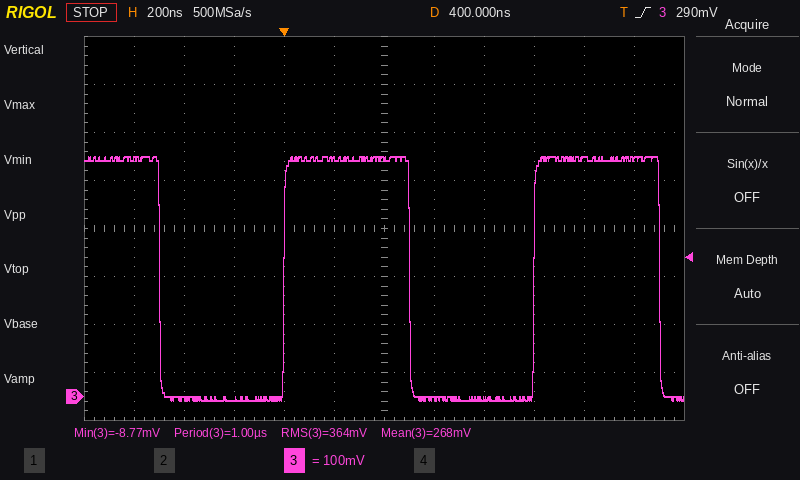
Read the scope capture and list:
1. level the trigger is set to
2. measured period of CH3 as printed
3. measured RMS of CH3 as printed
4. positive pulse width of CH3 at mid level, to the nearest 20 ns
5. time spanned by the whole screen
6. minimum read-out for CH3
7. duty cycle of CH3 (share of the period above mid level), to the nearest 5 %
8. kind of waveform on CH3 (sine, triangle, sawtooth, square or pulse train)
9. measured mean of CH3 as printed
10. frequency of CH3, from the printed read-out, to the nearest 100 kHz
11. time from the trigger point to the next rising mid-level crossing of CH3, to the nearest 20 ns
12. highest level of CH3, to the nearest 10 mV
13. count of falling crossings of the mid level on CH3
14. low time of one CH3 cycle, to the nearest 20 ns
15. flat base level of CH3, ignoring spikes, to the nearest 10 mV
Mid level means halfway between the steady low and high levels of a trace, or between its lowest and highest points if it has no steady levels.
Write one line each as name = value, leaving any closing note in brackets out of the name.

level the trigger is set to = 290 mV
measured period of CH3 as printed = 1.00 µs
measured RMS of CH3 as printed = 364 mV
positive pulse width of CH3 at mid level, to the nearest 20 ns = 500 ns
time spanned by the whole screen = 2.4 µs
minimum read-out for CH3 = -8.77 mV
duty cycle of CH3 (share of the period above mid level), to the nearest 5 % = 50 %
kind of waveform on CH3 = square
measured mean of CH3 as printed = 268 mV
frequency of CH3, from the printed read-out, to the nearest 100 kHz = 1.0 MHz
time from the trigger point to the next rising mid-level crossing of CH3, to the nearest 20 ns = 1.00 µs
highest level of CH3, to the nearest 10 mV = 500 mV
count of falling crossings of the mid level on CH3 = 3
low time of one CH3 cycle, to the nearest 20 ns = 500 ns
flat base level of CH3, ignoring spikes, to the nearest 10 mV = -10 mV
